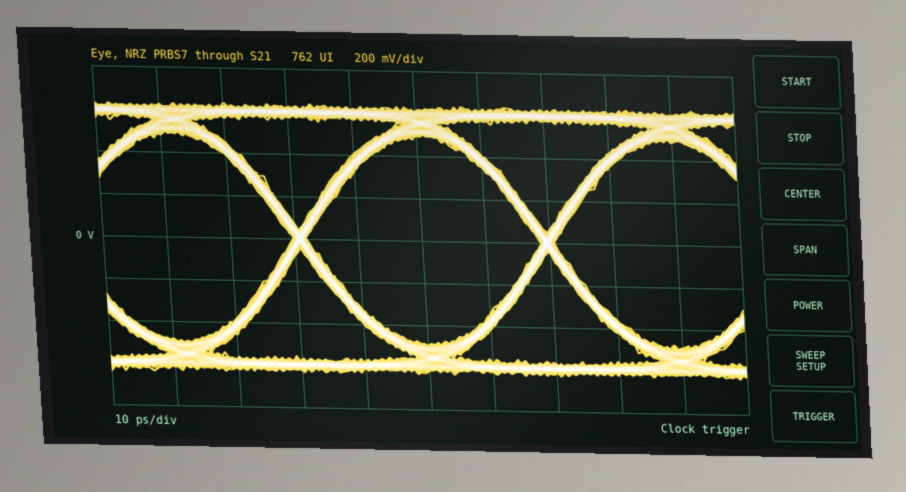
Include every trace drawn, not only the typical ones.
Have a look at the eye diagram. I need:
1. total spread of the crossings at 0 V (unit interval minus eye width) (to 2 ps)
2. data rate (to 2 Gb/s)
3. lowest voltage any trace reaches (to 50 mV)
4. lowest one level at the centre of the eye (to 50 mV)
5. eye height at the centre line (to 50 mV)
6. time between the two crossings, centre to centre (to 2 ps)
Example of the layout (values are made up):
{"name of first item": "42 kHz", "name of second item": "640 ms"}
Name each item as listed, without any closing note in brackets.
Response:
{"total spread of the crossings at 0 V (unit interval minus eye width)": "2 ps", "data rate": "26 Gb/s", "lowest voltage any trace reaches": "-650 mV", "lowest one level at the centre of the eye": "500 mV", "eye height at the centre line": "1.00 V", "time between the two crossings, centre to centre": "38 ps"}
